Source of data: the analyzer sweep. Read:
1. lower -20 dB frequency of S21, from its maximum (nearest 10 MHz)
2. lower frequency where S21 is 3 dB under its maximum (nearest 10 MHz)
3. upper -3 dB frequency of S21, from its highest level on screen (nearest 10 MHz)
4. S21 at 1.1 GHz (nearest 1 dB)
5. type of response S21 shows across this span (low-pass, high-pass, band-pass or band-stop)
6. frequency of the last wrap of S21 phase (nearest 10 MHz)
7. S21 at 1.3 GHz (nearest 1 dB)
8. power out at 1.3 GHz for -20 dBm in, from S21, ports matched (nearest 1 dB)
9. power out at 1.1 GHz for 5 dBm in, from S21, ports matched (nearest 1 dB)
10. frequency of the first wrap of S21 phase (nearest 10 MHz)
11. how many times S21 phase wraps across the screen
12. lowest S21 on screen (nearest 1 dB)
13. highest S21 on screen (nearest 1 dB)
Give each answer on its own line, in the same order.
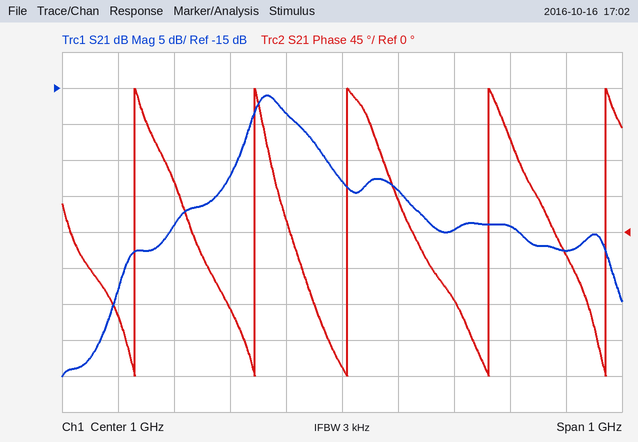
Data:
680 MHz
840 MHz
910 MHz
-29 dB
band-pass
1.47 GHz
-34 dB
-54 dBm
-24 dBm
630 MHz
5
-55 dB
-16 dB
